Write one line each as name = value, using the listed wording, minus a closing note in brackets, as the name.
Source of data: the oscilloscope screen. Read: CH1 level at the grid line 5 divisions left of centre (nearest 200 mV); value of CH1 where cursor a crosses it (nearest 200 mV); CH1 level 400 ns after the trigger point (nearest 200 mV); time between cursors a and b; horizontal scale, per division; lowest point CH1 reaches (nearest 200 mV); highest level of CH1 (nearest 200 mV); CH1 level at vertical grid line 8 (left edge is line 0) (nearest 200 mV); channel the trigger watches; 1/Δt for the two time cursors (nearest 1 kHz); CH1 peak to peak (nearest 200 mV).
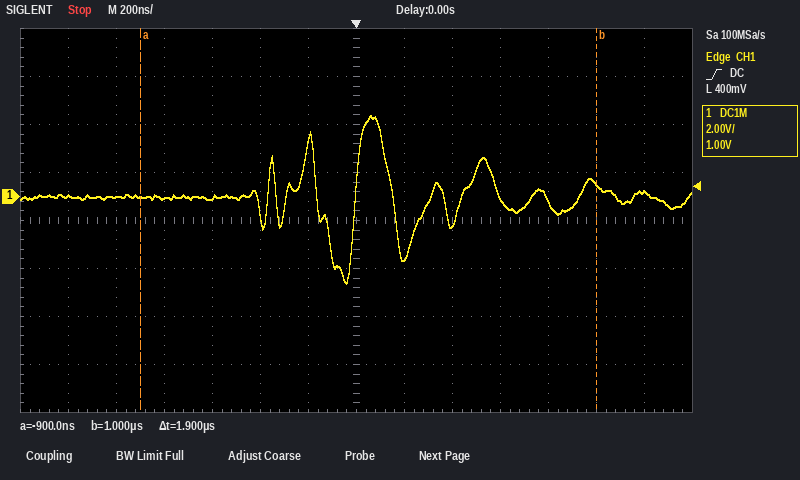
CH1 level at the grid line 5 divisions left of centre = 0.0 V
value of CH1 where cursor a crosses it = 0.0 V
CH1 level 400 ns after the trigger point = -1.2 V
time between cursors a and b = 1.9 µs
horizontal scale, per division = 200 ns
lowest point CH1 reaches = -3.6 V
highest level of CH1 = 3.4 V
CH1 level at vertical grid line 8 (left edge is line 0) = -2.6 V
channel the trigger watches = CH1
1/Δt for the two time cursors = 526 kHz
CH1 peak to peak = 7.0 V
